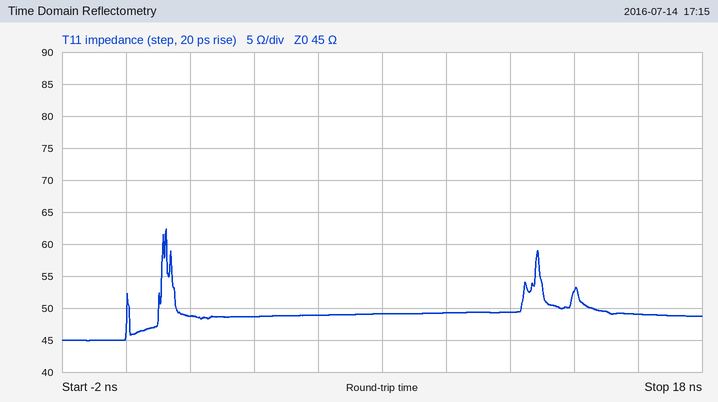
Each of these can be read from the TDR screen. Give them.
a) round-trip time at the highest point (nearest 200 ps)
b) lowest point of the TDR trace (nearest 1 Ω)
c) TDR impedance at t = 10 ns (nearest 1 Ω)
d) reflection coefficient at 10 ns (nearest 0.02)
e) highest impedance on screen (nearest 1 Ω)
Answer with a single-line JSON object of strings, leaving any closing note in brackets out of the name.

{"round-trip time at the highest point": "1.2 ns", "lowest point of the TDR trace": "45 Ω", "TDR impedance at t = 10 ns": "49 Ω", "reflection coefficient at 10 ns": "+0.04", "highest impedance on screen": "62 Ω"}
